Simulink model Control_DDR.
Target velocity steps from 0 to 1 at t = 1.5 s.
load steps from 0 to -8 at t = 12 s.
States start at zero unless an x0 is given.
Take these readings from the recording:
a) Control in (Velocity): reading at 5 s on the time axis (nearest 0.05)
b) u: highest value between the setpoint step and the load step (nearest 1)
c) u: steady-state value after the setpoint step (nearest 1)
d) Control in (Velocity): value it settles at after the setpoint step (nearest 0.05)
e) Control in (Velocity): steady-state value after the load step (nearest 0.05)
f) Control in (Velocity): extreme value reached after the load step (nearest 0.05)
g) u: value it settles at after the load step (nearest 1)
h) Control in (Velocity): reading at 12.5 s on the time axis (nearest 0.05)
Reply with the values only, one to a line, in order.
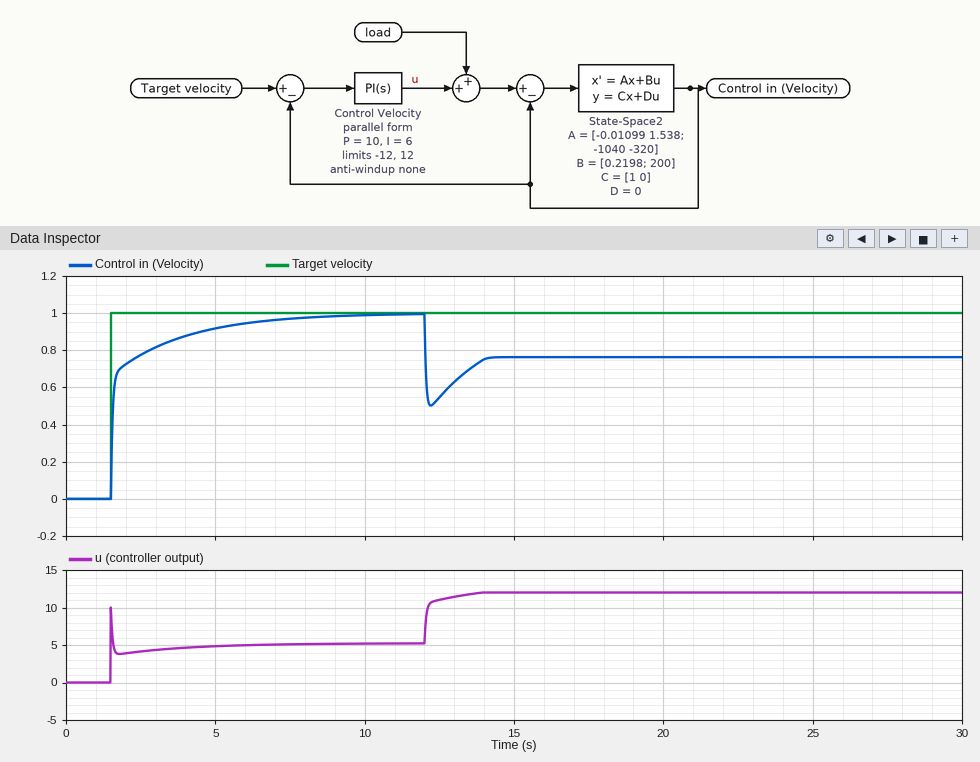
0.90
10
5
1.00
0.75
0.50
12
0.55
